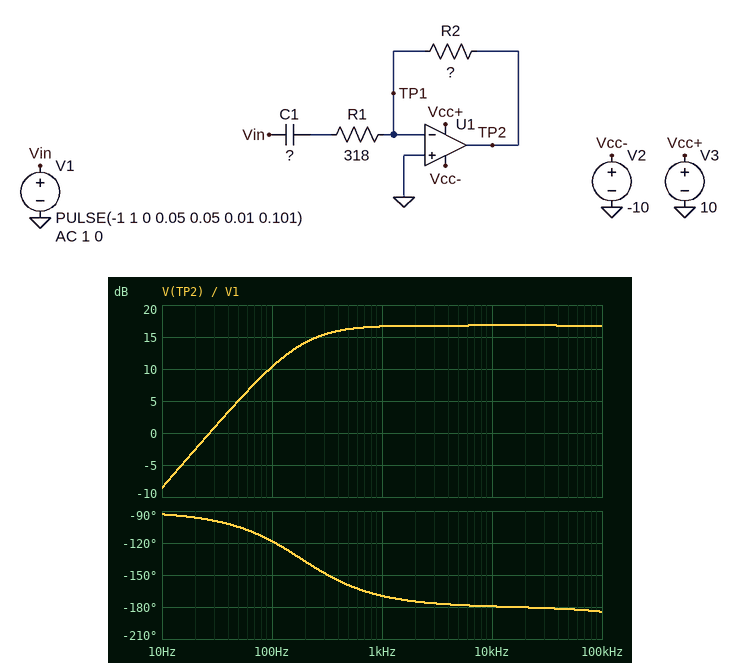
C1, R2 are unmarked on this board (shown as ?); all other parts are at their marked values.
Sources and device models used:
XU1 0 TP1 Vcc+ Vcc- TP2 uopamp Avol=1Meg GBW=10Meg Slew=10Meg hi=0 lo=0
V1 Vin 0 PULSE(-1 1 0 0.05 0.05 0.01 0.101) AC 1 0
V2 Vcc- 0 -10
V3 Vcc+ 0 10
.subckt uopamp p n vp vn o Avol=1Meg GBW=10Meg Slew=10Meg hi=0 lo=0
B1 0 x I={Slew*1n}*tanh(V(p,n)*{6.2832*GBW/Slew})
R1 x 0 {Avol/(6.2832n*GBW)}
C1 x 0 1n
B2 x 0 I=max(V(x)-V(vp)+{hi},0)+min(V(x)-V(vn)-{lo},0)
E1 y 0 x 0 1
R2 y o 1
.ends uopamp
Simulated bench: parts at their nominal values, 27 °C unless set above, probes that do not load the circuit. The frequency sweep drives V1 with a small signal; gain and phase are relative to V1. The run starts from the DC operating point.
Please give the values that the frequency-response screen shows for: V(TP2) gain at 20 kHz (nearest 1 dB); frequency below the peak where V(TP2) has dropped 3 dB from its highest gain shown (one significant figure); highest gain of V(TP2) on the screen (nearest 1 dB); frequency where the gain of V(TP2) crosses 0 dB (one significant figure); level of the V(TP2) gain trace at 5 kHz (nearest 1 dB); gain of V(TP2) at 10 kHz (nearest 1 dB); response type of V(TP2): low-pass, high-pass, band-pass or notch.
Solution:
17 dB
200 Hz
17 dB
30 Hz
17 dB
17 dB
high-pass
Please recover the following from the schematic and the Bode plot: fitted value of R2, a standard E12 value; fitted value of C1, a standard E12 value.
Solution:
2.2 kΩ
2.7 µF
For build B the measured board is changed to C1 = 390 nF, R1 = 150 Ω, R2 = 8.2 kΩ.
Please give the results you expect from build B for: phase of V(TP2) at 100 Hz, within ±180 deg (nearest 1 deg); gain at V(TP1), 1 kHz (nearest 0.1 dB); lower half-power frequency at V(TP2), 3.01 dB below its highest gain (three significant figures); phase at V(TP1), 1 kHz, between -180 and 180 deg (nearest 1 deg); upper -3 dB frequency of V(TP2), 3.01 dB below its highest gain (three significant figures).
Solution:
-92 deg
-54.5 dB
2.68 kHz
159 deg
182 kHz
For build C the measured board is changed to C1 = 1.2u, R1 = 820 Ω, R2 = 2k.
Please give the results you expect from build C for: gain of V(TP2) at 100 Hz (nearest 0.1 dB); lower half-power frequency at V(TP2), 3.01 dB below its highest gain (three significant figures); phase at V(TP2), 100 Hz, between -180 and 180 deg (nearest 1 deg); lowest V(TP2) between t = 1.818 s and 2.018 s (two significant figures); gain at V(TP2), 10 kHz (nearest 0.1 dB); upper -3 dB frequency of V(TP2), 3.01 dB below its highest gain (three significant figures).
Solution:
2.2 dB
162 Hz
-122 deg
-96 mV
7.7 dB
2.91 MHz
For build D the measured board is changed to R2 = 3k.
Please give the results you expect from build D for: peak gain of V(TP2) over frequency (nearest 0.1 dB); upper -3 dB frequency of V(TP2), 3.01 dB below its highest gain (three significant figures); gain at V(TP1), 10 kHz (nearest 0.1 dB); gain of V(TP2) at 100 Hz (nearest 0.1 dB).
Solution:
19.5 dB
958 kHz
-40.5 dB
13.0 dB
